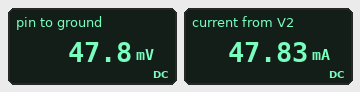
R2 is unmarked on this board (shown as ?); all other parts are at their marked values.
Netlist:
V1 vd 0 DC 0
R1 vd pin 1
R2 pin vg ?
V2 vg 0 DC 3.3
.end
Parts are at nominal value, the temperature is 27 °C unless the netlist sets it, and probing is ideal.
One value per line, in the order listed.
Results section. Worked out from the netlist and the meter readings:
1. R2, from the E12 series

68 Ω
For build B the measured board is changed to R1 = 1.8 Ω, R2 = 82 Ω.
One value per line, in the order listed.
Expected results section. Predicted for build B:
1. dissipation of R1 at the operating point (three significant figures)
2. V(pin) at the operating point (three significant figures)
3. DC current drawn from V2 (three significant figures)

2.79 mW
70.9 mV
39.4 mA
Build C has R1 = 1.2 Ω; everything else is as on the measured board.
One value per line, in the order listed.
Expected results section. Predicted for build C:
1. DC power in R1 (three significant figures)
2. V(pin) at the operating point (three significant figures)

2.73 mW
57.2 mV
